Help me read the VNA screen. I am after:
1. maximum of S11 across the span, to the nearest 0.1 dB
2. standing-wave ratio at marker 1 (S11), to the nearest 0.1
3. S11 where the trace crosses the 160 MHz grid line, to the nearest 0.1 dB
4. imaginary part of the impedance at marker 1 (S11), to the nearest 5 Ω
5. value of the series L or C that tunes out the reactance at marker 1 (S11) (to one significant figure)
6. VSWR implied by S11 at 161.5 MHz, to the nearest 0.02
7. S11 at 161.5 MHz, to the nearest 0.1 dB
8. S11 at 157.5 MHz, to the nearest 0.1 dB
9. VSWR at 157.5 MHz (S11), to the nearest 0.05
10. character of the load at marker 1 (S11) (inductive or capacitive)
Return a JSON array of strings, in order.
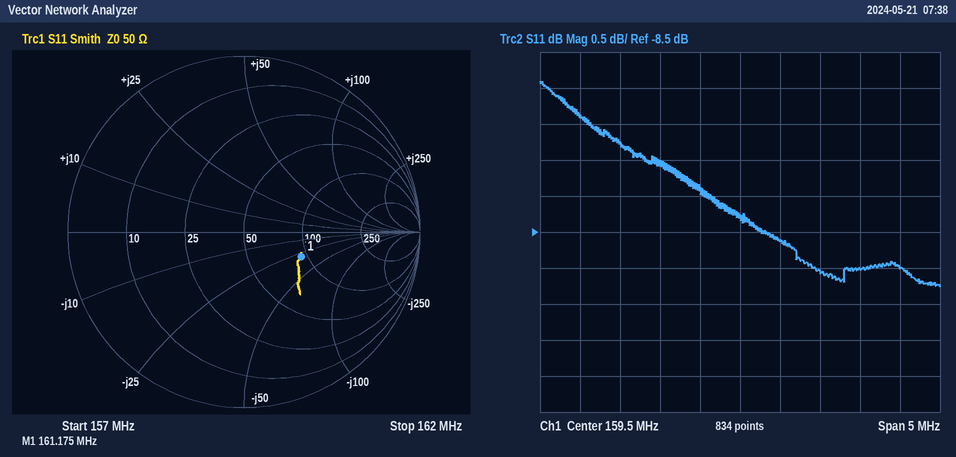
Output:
["-6.4 dB", "2.1", "-8.6 dB", "-30 Ω", "30 nH", "2.10", "-9.0 dB", "-6.9 dB", "2.65", "capacitive"]
